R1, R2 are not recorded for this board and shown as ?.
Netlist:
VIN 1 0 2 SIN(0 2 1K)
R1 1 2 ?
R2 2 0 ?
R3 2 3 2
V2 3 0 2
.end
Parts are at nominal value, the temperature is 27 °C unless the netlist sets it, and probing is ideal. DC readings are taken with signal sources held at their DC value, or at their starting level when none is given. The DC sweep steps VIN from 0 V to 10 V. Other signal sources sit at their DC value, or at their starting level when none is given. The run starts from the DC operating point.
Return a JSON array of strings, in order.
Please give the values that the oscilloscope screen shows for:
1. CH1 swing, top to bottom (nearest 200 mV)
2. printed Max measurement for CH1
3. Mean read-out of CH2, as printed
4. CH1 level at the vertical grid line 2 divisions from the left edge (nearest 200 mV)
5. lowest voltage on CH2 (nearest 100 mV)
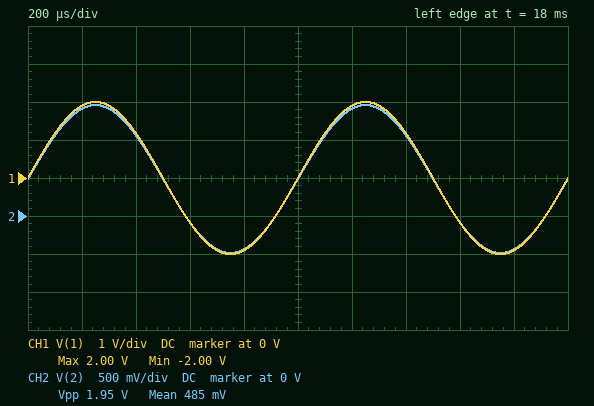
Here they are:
["4.0 V", "2.00 V", "485 mV", "1.2 V", "-500 mV"]
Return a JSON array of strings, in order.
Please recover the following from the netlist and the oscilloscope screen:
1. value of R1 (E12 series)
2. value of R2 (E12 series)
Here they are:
["1 Ω", "1.8 Ω"]
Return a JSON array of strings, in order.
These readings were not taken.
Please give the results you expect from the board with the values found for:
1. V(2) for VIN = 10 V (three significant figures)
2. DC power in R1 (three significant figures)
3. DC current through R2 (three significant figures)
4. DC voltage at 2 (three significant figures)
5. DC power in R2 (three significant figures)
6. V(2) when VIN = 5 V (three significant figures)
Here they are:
["5.35 V", "292 mW", "811 mA", "1.46 V", "1.18 W", "2.92 V"]
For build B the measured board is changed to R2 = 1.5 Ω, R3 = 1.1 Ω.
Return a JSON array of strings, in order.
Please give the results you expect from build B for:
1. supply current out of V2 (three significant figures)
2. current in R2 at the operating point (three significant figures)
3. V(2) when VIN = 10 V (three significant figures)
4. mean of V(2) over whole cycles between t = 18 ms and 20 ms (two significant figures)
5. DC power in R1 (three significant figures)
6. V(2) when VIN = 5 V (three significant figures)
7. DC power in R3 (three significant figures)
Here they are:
["471 mA", "988 mA", "4.59 V", "710 mV", "268 mW", "2.65 V", "244 mW"]
